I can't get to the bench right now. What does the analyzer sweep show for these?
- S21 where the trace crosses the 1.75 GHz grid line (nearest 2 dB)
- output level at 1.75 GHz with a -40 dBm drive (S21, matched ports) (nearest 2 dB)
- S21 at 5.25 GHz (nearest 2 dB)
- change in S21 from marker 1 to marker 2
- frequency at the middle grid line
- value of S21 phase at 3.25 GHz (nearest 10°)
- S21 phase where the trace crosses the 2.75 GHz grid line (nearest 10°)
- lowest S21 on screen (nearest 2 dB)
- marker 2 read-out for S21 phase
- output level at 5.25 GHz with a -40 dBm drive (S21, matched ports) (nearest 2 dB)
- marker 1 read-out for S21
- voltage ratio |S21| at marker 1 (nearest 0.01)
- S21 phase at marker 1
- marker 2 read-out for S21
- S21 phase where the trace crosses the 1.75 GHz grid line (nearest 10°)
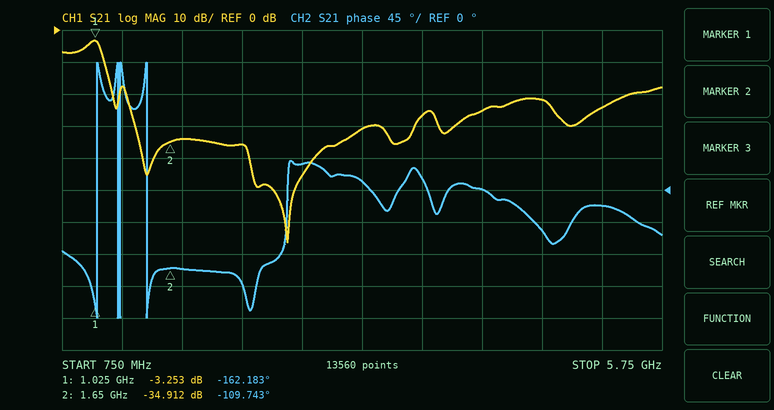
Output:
-34 dB
-74 dBm
-24 dB
-31.659 dB
3.25 GHz
10°
40°
-66 dB
-109.743°
-64 dBm
-3.253 dB
0.69
-162.183°
-34.912 dB
-110°
